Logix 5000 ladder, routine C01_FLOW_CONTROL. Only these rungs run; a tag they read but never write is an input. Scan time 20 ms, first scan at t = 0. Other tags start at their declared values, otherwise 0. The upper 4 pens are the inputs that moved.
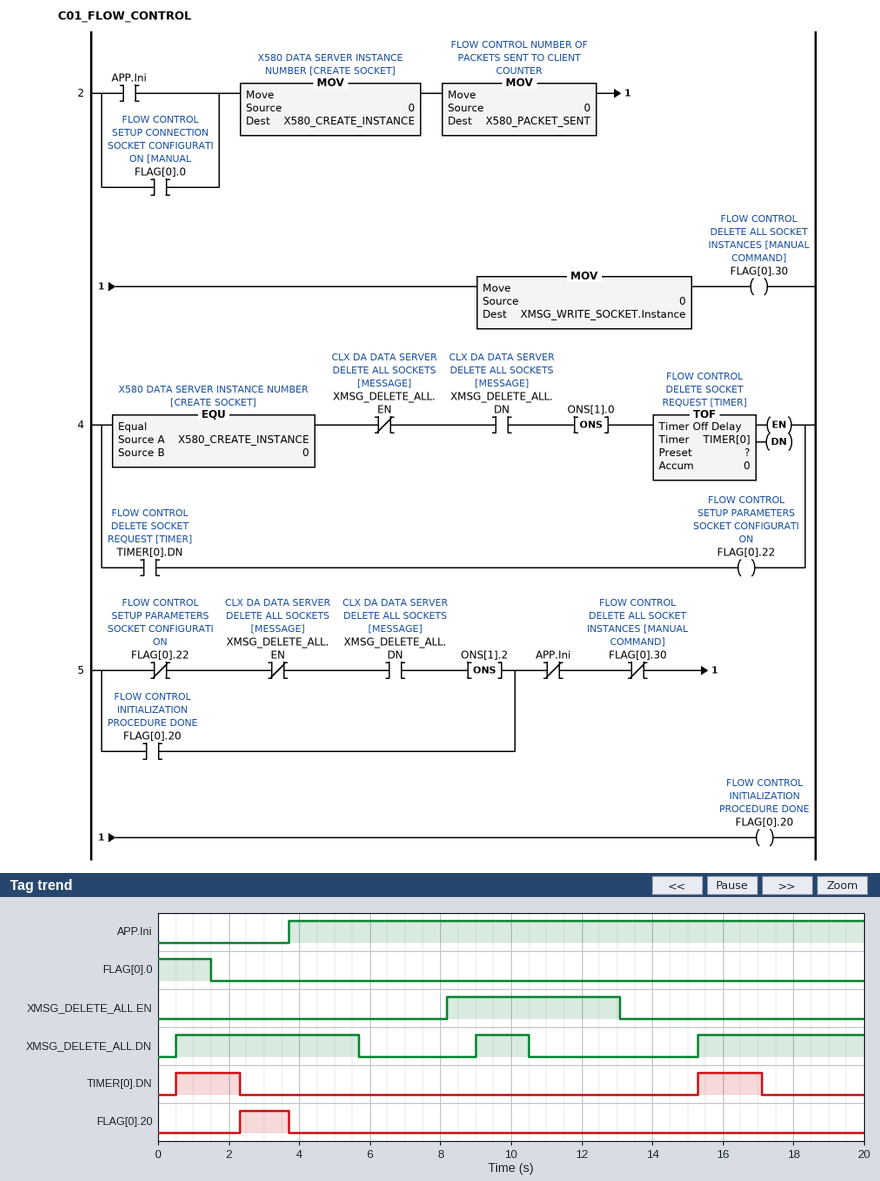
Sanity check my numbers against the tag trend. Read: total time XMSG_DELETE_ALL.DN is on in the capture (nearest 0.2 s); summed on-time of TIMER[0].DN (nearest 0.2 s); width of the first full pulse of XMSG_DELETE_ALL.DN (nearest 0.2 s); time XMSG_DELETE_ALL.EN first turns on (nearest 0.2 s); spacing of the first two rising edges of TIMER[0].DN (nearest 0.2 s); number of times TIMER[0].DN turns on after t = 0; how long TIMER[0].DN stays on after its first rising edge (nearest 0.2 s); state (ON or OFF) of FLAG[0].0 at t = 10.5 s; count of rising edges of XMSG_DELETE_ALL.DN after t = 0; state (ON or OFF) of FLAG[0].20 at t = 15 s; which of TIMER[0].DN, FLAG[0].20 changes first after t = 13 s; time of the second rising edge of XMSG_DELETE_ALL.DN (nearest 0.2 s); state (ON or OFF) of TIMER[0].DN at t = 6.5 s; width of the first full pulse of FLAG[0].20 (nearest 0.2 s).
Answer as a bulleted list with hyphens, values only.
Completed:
- 11.4 s
- 3.6 s
- 5.2 s
- 8.2 s
- 14.8 s
- 2
- 1.8 s
- OFF
- 3
- OFF
- TIMER[0].DN
- 9.0 s
- OFF
- 1.4 s
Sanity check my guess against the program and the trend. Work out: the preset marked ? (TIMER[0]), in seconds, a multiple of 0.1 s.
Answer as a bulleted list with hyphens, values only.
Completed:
- 1.8 s
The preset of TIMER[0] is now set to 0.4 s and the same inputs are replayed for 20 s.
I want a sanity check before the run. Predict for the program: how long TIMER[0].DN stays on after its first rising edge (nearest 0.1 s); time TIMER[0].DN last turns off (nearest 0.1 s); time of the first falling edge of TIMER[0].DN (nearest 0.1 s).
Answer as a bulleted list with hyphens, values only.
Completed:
- 0.4 s
- 15.7 s
- 0.9 s
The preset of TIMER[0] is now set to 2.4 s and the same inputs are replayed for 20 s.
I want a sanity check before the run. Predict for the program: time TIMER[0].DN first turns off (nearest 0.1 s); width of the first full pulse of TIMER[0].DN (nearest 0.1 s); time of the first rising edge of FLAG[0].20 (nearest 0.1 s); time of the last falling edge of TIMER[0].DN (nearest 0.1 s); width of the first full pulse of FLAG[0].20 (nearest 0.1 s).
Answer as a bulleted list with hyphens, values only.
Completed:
- 2.9 s
- 2.4 s
- 2.9 s
- 17.7 s
- 0.8 s
